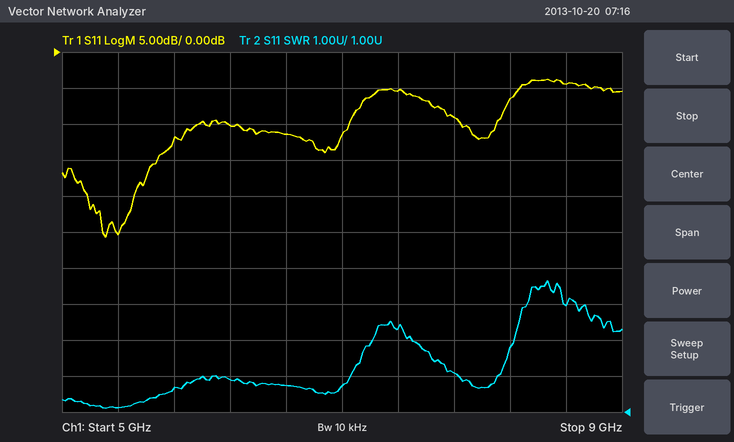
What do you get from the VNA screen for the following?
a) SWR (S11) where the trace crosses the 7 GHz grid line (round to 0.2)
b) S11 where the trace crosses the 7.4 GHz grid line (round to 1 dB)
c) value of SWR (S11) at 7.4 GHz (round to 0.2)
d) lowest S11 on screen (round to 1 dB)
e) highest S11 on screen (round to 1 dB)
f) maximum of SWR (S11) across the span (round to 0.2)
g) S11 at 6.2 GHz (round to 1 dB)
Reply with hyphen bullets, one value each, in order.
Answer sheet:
- 1.8
- -5 dB
- 3.4
- -26 dB
- -4 dB
- 4.6
- -10 dB
